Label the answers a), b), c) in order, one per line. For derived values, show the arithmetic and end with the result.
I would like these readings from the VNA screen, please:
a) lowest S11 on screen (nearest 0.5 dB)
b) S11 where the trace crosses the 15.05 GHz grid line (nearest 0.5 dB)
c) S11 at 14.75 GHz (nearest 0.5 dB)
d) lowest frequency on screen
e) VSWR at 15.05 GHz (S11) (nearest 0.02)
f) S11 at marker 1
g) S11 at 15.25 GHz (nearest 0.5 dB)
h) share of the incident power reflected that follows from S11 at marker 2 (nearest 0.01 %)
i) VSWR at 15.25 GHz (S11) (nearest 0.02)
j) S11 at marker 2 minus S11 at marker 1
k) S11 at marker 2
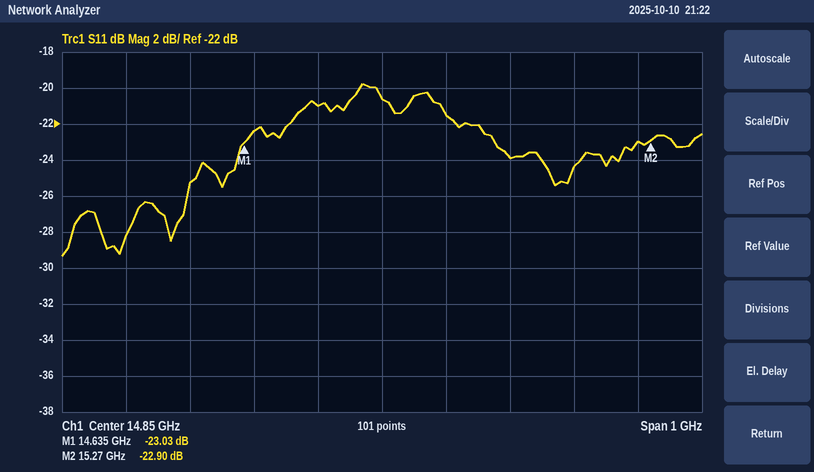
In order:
a) -29.5 dB
b) -24.0 dB
c) -21.0 dB
d) 14.35 GHz
e) |Γ| = 10^(-24/20) = 0.0631; VSWR = (1 + 0.0631)/(1 − 0.0631) ≈ 1.13, so 1.14 to the nearest 0.02
f) -23.03 dB
g) -23.0 dB
h) 10^(-22.9/10) ≈ 0.51 %
i) |Γ| = 10^(-23/20) = 0.0708; VSWR = (1 + 0.0708)/(1 − 0.0708) ≈ 1.15, so 1.16 to the nearest 0.02
j) -22.9 − (-23.03) = 0.13 dB
k) -22.90 dB
